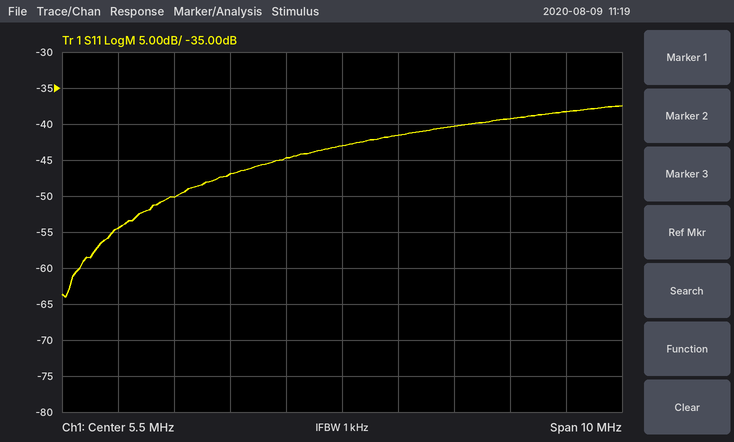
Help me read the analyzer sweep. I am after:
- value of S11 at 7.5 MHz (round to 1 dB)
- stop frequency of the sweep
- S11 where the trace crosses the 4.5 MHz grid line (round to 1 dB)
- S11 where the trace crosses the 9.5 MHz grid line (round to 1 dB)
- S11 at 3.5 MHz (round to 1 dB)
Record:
-40 dB
10.5 MHz
-45 dB
-38 dB
-47 dB
